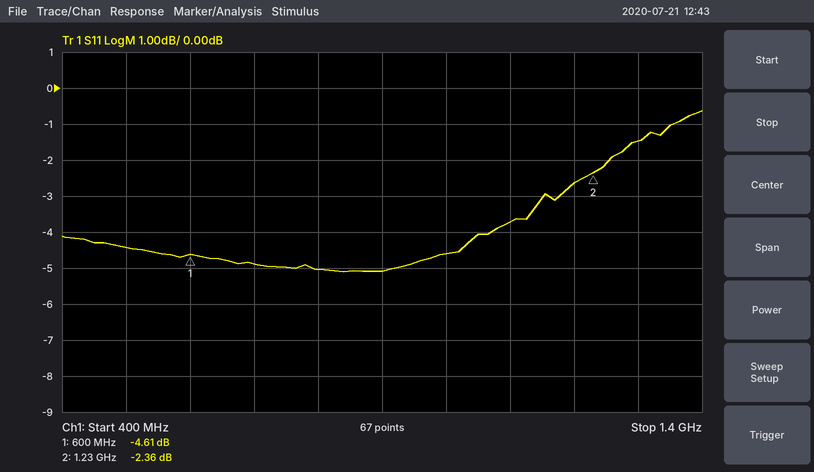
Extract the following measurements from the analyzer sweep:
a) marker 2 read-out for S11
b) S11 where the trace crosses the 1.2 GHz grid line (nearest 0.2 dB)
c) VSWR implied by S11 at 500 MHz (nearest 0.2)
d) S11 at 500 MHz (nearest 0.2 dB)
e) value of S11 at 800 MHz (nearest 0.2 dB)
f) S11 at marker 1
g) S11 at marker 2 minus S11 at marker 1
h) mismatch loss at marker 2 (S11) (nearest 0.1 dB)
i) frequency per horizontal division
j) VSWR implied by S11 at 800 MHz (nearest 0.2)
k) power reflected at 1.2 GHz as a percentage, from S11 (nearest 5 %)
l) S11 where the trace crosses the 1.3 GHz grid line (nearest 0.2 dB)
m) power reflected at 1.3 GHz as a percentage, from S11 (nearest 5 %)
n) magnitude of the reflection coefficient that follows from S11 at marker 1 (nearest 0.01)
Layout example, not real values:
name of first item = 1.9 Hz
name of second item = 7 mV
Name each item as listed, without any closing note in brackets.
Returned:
marker 2 read-out for S11 = -2.36 dB
S11 where the trace crosses the 1.2 GHz grid line = -2.6 dB
VSWR implied by S11 at 500 MHz = 4.0
S11 at 500 MHz = -4.4 dB
value of S11 at 800 MHz = -5.0 dB
S11 at marker 1 = -4.61 dB
S11 at marker 2 minus S11 at marker 1 = 2.25 dB
mismatch loss at marker 2 (S11) = 3.8 dB
frequency per horizontal division = 100 MHz
VSWR implied by S11 at 800 MHz = 3.6
power reflected at 1.2 GHz as a percentage, from S11 = 55 %
S11 where the trace crosses the 1.3 GHz grid line = -1.4 dB
power reflected at 1.3 GHz as a percentage, from S11 = 70 %
magnitude of the reflection coefficient that follows from S11 at marker 1 = 0.59
